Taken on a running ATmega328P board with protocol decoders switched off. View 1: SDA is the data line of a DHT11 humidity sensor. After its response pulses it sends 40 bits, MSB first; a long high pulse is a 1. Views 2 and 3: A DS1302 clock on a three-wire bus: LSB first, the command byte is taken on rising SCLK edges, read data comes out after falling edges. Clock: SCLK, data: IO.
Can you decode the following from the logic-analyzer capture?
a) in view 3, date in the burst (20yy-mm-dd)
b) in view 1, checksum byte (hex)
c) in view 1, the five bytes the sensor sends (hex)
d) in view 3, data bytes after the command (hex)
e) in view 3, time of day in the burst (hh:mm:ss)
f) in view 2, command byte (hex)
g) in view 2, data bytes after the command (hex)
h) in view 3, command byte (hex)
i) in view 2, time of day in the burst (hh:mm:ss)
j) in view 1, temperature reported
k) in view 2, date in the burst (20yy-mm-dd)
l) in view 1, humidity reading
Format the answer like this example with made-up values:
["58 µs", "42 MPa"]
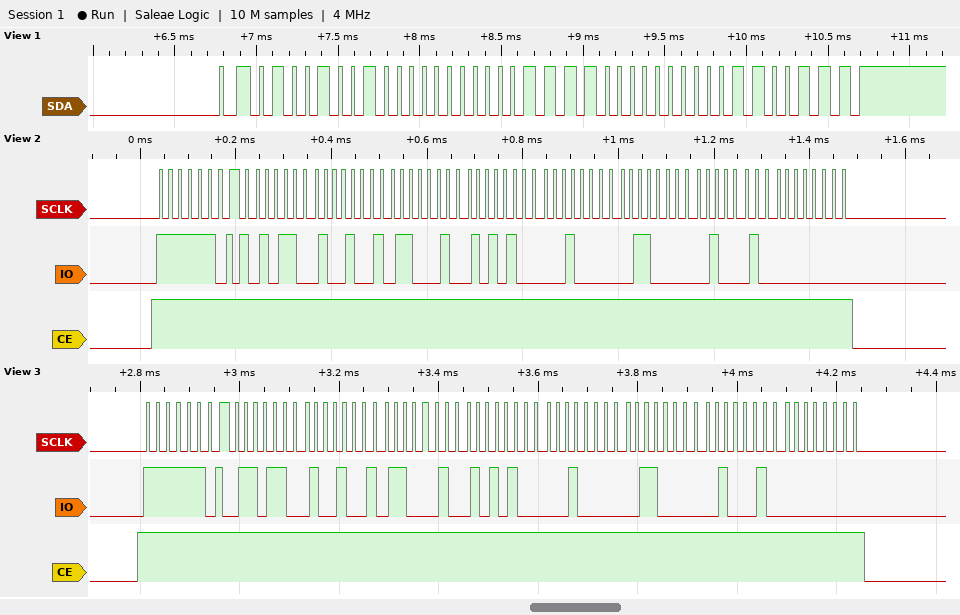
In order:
["2022-04-15", "0x67", "49 00 1E 00 67", "36 49 23 15 04 06 22 00", "23:49:36", "0xBF", "35 49 23 15 04 06 22 00", "0xBF", "23:49:35", "30.0 °C", "2022-04-15", "73 %"]
